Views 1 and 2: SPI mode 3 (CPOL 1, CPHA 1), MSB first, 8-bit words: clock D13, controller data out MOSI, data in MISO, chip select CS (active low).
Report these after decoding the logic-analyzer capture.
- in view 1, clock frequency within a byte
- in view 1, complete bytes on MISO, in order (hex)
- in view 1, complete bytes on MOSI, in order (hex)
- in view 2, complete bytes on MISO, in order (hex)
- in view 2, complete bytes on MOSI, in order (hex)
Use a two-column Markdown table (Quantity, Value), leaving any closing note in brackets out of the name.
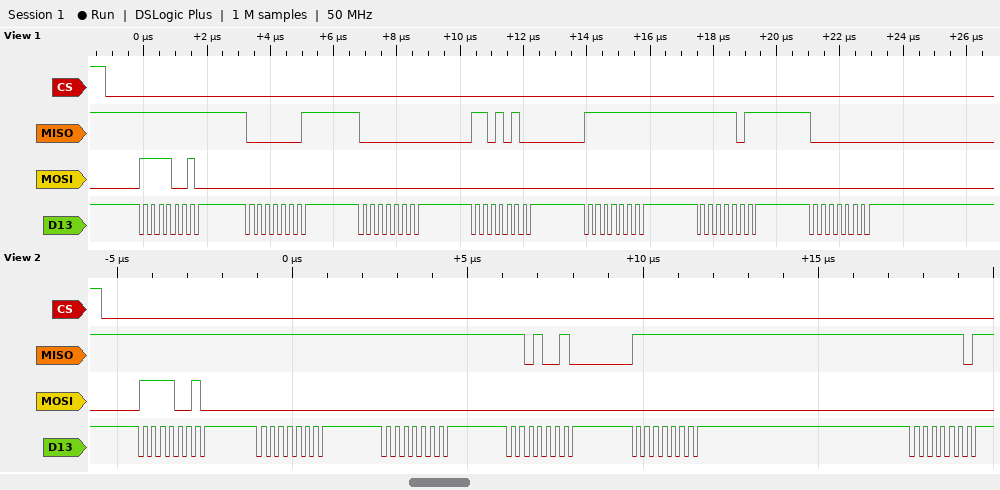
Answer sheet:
| Quantity | Value |
|---|---|
| in view 1, clock frequency within a byte | 4 MHz |
| in view 1, complete bytes on MISO, in order | FF 01 00 D4 FF FB 00 |
| in view 1, complete bytes on MOSI, in order | F2 00 00 00 00 00 00 |
| in view 2, complete bytes on MISO, in order | 0xFF 0xFF 0xFF 0xD2 0xFF 0xFD |
| in view 2, complete bytes on MOSI, in order | 0xF2 0x00 0x00 0x00 0x00 0x00 |
